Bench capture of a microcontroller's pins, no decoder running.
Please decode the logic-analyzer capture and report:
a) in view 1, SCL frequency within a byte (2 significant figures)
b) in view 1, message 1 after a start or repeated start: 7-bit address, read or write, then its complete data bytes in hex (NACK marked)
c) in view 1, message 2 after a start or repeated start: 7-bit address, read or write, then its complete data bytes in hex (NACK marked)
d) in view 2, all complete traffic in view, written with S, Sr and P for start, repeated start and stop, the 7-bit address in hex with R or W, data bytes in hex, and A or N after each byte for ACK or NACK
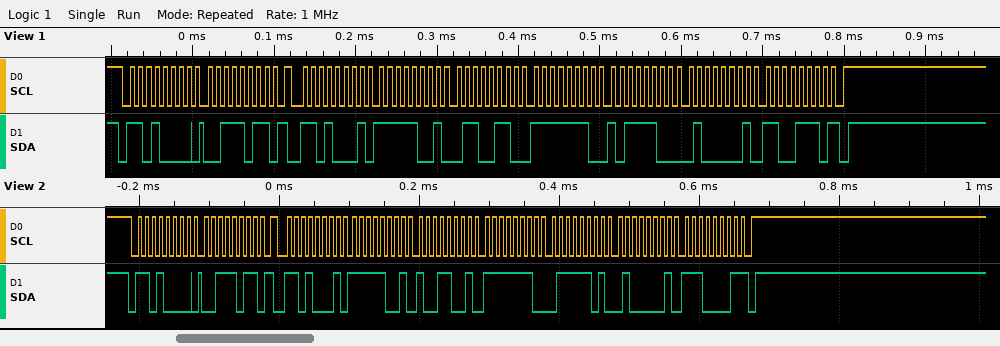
100 kHz
0x68 write: 3B
0x68 read: F9 66 FE BC 41 CE NACK
S 68W A 3B A Sr 68R A F9 A 99 A FE A 7D A 41 A E1 N P
